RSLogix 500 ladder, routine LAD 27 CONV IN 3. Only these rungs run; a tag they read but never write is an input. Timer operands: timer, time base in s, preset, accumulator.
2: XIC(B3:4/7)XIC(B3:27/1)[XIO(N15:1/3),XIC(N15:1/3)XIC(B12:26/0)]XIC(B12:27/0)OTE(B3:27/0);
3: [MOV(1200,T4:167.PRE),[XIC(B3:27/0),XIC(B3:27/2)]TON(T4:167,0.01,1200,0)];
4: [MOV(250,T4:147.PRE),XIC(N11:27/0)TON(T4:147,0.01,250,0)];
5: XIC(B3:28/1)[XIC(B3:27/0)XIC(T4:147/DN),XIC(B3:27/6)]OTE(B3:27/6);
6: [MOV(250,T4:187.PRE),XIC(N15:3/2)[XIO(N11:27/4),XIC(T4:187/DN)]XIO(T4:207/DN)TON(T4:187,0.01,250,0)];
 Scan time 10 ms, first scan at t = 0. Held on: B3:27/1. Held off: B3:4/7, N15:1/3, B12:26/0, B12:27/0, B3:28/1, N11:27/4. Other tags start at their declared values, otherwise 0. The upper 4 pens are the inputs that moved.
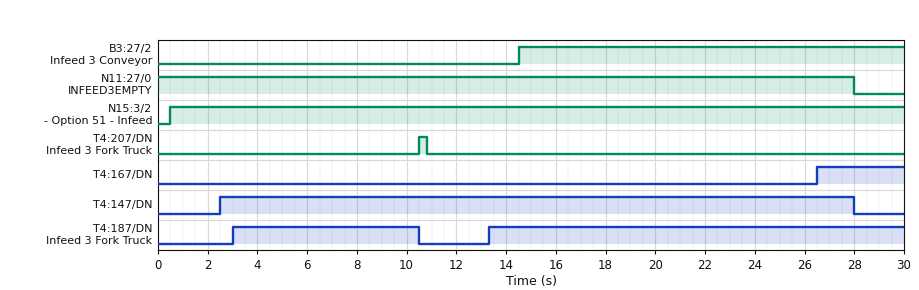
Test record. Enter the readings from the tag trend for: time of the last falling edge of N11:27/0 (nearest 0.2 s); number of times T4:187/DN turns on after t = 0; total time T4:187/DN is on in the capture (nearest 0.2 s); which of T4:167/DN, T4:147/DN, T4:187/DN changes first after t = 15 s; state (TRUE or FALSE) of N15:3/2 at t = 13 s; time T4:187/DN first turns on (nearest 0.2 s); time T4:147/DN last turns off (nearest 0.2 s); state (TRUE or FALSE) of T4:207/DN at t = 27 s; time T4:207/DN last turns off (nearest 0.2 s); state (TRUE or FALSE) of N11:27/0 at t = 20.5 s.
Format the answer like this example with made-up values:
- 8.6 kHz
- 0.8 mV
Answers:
- 28.0 s
- 2
- 24.2 s
- T4:167/DN
- TRUE
- 3.0 s
- 28.0 s
- FALSE
- 10.8 s
- TRUE
